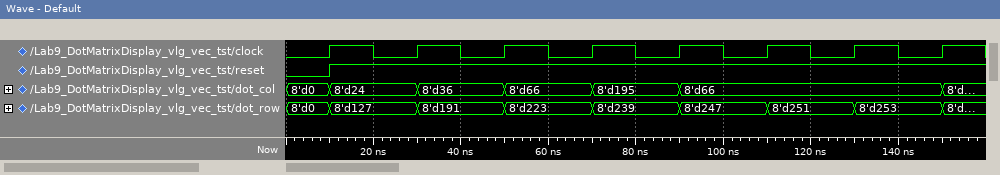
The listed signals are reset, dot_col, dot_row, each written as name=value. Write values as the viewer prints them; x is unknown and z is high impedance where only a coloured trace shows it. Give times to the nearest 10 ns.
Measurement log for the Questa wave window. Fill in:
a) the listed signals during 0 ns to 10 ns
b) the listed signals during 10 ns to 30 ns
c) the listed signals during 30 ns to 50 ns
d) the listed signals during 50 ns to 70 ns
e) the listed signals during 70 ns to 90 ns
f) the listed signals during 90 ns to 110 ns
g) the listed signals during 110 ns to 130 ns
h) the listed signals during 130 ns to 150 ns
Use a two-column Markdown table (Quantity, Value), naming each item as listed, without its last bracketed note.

| Quantity | Value |
|---|---|
| the listed signals during 0 ns to 10 ns | reset=0, dot_col=8'd0, dot_row=8'd0 |
| the listed signals during 10 ns to 30 ns | reset=1, dot_col=8'd24, dot_row=8'd127 |
| the listed signals during 30 ns to 50 ns | reset=1, dot_col=8'd36, dot_row=8'd191 |
| the listed signals during 50 ns to 70 ns | reset=1, dot_col=8'd66, dot_row=8'd223 |
| the listed signals during 70 ns to 90 ns | reset=1, dot_col=8'd195, dot_row=8'd239 |
| the listed signals during 90 ns to 110 ns | reset=1, dot_col=8'd66, dot_row=8'd247 |
| the listed signals during 110 ns to 130 ns | reset=1, dot_col=8'd66, dot_row=8'd251 |
| the listed signals during 130 ns to 150 ns | reset=1, dot_col=8'd66, dot_row=8'd253 |
